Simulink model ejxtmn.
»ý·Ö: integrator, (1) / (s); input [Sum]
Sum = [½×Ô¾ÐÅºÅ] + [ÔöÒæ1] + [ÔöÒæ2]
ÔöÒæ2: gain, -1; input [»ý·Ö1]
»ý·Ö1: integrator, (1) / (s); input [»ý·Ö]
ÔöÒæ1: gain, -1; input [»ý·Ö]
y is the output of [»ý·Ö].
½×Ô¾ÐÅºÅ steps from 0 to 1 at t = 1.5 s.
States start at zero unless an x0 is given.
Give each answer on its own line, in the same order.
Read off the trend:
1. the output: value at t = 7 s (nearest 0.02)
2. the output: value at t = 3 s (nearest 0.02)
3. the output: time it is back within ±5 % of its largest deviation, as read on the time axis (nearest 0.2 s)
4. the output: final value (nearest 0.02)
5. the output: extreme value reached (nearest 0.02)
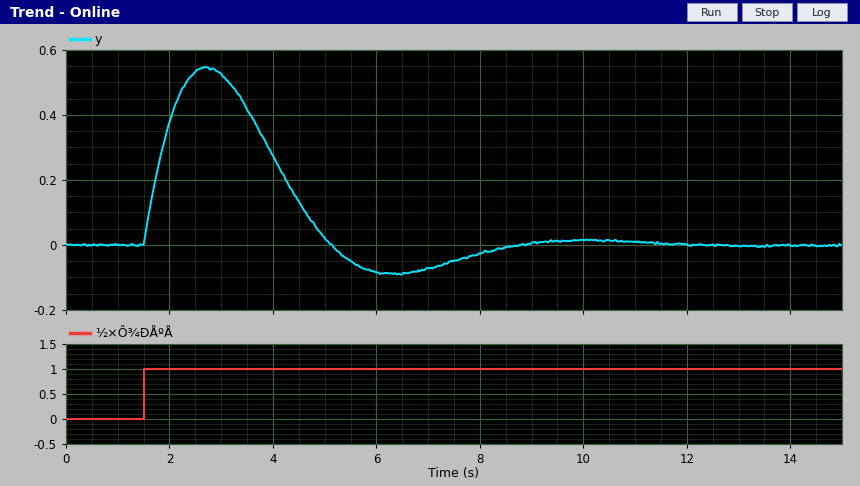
-0.08
0.52
8.0 s
0.00
0.54
